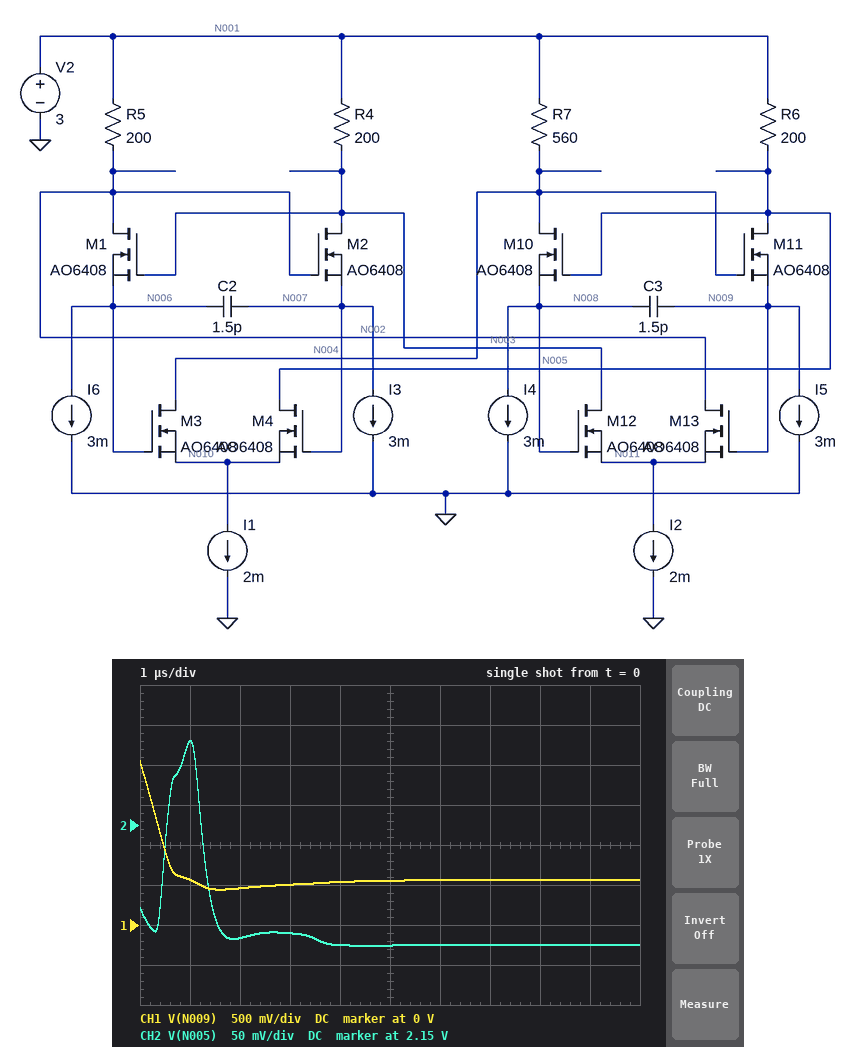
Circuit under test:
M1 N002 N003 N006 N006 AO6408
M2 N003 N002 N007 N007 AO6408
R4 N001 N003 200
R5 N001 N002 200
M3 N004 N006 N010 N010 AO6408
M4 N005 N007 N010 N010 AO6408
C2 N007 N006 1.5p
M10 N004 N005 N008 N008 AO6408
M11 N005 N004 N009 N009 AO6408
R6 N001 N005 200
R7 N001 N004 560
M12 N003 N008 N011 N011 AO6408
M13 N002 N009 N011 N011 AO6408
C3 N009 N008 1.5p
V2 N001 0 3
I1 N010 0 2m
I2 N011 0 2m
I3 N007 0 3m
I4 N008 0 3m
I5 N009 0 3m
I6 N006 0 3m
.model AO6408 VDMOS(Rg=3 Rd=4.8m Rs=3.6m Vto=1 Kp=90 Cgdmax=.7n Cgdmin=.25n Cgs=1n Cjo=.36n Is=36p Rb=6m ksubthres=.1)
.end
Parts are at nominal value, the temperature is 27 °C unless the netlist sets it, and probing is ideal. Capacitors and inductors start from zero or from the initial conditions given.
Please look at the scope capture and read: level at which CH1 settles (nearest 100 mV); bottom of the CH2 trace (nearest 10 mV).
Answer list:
600 mV
2.00 V
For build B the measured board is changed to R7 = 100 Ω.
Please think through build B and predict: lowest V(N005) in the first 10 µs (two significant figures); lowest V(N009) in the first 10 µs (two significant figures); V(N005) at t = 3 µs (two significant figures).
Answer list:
2.1 V
1.7 V
2.4 V
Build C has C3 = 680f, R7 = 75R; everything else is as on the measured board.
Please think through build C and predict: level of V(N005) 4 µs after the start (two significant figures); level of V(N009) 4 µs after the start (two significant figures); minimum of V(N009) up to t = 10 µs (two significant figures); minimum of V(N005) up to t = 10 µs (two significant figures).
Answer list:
2.4 V
1.9 V
1.8 V
2.1 V
